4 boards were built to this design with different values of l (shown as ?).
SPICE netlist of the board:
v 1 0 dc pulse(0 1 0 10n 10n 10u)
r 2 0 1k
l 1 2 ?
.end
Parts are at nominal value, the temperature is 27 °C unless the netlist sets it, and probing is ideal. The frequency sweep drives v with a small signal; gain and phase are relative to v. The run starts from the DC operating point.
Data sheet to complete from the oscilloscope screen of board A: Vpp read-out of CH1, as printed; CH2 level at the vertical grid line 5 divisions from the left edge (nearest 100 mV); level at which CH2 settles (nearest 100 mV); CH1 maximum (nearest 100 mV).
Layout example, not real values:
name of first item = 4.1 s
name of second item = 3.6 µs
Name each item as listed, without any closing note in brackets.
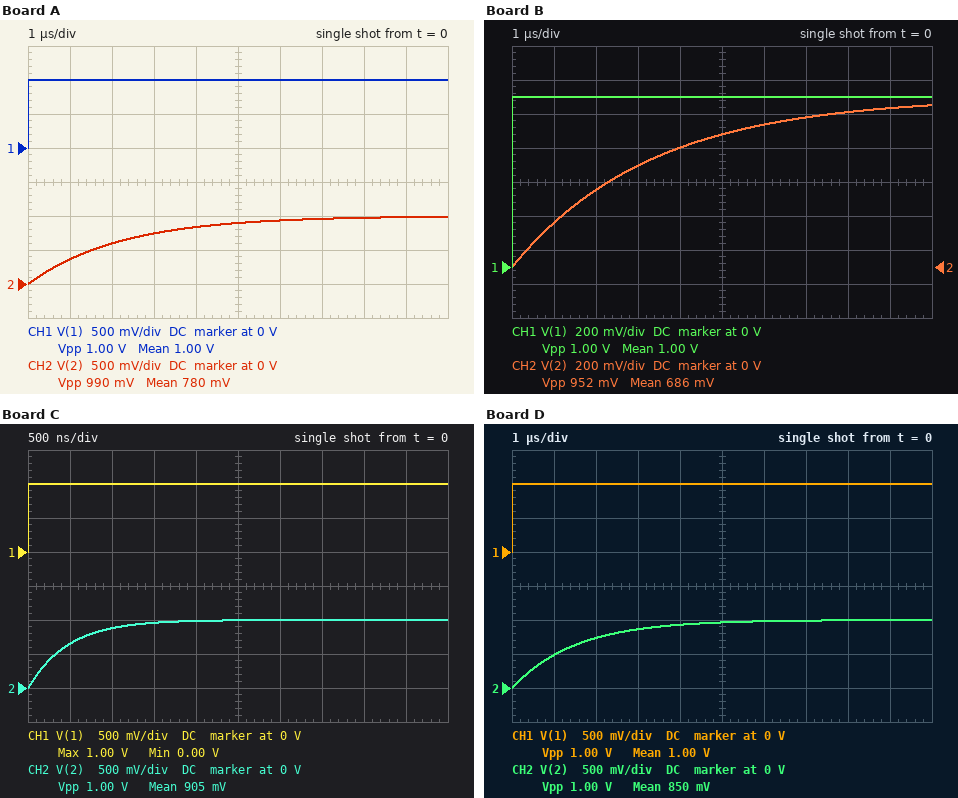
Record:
Vpp read-out of CH1, as printed = 1.00 V
CH2 level at the vertical grid line 5 divisions from the left edge = 900 mV
level at which CH2 settles = 1.0 V
CH1 maximum = 1.0 V
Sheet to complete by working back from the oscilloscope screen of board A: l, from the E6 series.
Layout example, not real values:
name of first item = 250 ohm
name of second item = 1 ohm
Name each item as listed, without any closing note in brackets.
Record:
l, from the E6 series = 2.2 mH
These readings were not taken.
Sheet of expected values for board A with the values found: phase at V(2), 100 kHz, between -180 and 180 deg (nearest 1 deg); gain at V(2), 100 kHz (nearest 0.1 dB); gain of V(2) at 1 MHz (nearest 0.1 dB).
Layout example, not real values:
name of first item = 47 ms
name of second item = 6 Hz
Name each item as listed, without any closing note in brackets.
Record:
phase at V(2), 100 kHz, between -180 and 180 deg = -54 deg
gain at V(2), 100 kHz = -4.6 dB
gain of V(2) at 1 MHz = -22.8 dB
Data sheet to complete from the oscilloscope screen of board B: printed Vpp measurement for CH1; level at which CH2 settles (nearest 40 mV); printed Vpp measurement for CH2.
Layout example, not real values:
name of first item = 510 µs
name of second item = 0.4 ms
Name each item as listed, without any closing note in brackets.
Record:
printed Vpp measurement for CH1 = 1.00 V
level at which CH2 settles = 960 mV
printed Vpp measurement for CH2 = 952 mV
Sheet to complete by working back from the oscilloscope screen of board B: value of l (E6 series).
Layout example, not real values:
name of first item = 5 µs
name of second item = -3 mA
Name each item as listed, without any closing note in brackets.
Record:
value of l = 3.3 mH
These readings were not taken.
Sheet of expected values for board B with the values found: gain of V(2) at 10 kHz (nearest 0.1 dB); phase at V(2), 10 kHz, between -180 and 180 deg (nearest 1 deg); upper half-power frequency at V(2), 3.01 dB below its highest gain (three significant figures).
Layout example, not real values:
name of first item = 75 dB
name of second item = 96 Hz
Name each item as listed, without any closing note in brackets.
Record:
gain of V(2) at 10 kHz = -0.2 dB
phase at V(2), 10 kHz, between -180 and 180 deg = -12 deg
upper half-power frequency at V(2), 3.01 dB below its highest gain = 48.2 kHz
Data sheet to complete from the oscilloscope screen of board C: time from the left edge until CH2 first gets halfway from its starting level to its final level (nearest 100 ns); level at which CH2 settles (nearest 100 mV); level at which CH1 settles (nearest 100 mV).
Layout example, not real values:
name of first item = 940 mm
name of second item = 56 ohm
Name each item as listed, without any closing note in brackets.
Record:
time from the left edge until CH2 first gets halfway from its starting level to its final level = 300 ns
level at which CH2 settles = 1.0 V
level at which CH1 settles = 1.0 V
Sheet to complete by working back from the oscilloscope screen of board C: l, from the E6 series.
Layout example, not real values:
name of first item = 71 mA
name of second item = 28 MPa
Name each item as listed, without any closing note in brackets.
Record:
l, from the E6 series = 470 µH
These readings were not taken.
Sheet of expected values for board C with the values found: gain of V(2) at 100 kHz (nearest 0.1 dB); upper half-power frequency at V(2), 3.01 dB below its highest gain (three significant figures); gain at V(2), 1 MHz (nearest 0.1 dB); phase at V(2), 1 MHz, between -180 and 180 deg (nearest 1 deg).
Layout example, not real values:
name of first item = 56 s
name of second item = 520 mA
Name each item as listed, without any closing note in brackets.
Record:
gain of V(2) at 100 kHz = -0.4 dB
upper half-power frequency at V(2), 3.01 dB below its highest gain = 339 kHz
gain at V(2), 1 MHz = -9.9 dB
phase at V(2), 1 MHz, between -180 and 180 deg = -71 deg
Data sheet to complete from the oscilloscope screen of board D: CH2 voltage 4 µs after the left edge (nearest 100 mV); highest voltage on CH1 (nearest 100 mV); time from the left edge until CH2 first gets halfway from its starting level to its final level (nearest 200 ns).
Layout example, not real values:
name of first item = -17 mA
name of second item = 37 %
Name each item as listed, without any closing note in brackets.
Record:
CH2 voltage 4 µs after the left edge = 900 mV
highest voltage on CH1 = 1.0 V
time from the left edge until CH2 first gets halfway from its starting level to its final level = 1.0 µs
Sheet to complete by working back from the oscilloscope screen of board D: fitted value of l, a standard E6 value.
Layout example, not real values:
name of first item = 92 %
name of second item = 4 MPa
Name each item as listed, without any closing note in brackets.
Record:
fitted value of l, a standard E6 value = 1.5 mH
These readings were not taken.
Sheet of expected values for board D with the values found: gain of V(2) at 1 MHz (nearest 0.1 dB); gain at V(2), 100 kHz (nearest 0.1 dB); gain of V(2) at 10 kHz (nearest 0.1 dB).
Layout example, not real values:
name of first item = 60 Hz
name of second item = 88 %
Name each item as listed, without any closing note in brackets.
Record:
gain of V(2) at 1 MHz = -19.5 dB
gain at V(2), 100 kHz = -2.8 dB
gain of V(2) at 10 kHz = 0 dB
